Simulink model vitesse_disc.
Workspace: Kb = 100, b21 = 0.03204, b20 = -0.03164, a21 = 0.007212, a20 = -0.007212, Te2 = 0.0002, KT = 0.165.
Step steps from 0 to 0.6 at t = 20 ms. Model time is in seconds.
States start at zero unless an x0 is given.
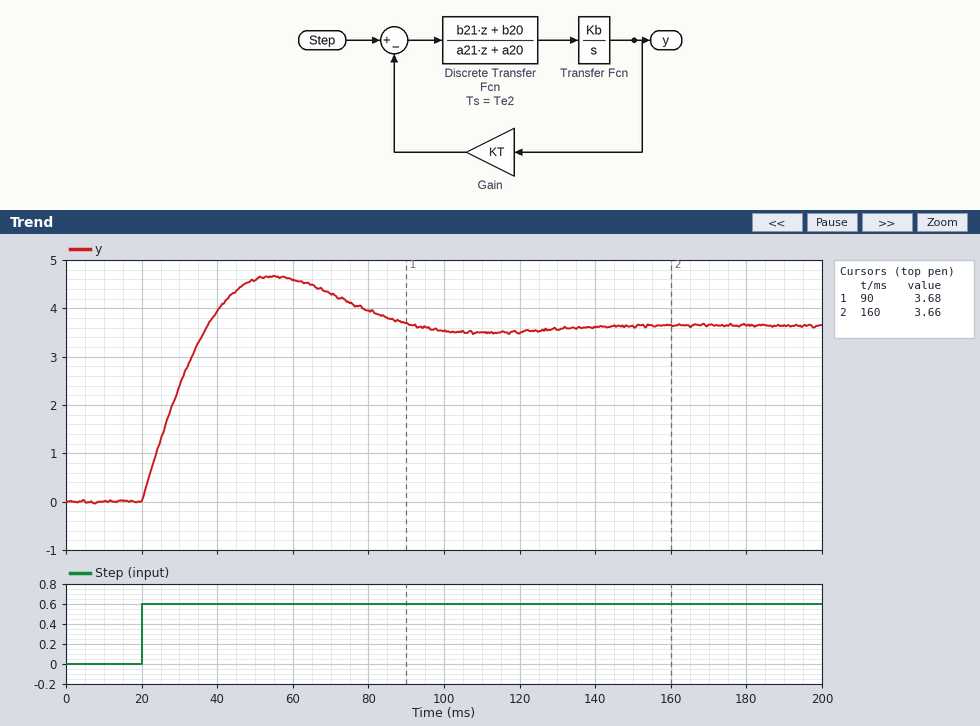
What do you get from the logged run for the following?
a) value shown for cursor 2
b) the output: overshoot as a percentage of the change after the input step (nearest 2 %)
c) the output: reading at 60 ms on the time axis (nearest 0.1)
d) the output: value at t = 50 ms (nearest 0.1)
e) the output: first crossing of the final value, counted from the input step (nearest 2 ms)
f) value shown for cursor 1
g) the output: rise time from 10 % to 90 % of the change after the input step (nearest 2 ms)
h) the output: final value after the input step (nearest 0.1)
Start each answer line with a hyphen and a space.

- 3.66
- 28 %
- 4.6
- 4.6
- 18 ms
- 3.68
- 14 ms
- 3.6
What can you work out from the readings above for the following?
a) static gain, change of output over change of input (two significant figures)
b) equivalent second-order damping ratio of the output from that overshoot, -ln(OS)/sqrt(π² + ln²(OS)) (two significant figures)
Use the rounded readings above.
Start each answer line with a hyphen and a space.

- 6.0
- 0.38
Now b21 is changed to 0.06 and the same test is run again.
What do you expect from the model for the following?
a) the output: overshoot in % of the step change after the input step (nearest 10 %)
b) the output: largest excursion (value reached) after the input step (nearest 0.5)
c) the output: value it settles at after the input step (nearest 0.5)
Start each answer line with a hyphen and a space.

- 80 %
- 6.5
- 3.5
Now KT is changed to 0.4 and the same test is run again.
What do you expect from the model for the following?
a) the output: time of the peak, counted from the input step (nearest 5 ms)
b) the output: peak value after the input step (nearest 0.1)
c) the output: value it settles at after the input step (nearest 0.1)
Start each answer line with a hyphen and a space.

- 20 ms
- 1.8
- 1.5
